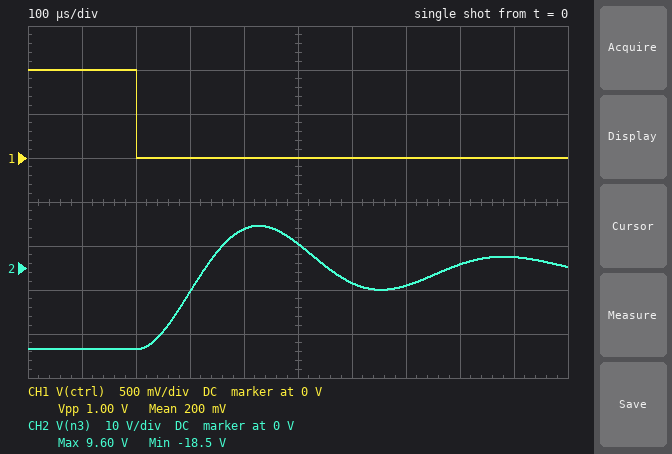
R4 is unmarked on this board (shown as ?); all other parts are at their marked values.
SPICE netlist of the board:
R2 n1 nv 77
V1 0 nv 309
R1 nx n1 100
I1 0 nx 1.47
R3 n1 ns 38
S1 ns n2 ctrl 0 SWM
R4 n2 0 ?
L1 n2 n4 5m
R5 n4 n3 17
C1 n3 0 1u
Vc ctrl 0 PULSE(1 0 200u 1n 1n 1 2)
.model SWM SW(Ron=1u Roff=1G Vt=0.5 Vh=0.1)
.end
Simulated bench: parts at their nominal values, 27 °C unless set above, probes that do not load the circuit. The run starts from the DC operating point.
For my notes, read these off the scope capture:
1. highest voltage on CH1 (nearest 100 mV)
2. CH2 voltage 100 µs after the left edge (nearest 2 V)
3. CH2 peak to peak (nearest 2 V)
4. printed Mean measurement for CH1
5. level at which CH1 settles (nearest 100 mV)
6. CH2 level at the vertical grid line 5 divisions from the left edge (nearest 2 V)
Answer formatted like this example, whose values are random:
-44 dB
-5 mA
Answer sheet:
1.0 V
-18 V
28 V
200 mV
0 V
6 V
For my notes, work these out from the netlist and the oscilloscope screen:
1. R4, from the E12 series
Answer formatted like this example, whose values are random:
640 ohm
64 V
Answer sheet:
12 Ω
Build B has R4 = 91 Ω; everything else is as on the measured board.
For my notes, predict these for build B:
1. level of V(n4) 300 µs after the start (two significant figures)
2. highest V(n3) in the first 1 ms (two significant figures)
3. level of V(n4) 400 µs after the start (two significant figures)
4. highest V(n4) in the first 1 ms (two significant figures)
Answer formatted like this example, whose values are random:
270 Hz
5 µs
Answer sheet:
-37 V
2.1 V
-5.3 V
2.2 V
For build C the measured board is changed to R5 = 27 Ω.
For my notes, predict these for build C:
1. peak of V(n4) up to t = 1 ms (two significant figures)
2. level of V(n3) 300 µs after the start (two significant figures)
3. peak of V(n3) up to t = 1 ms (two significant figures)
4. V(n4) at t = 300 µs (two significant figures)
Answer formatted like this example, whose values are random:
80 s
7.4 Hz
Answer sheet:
8.1 V
-6.1 V
7.5 V
-1.3 V
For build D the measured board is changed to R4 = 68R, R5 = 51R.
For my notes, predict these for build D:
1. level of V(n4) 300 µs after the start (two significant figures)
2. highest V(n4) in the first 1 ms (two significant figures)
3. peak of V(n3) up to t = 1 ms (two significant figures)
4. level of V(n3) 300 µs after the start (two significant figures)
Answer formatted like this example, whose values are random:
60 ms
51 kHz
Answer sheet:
-19 V
1.0 V
550 mV
-40 V
